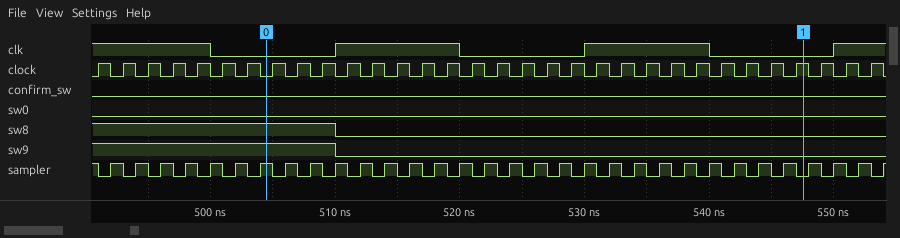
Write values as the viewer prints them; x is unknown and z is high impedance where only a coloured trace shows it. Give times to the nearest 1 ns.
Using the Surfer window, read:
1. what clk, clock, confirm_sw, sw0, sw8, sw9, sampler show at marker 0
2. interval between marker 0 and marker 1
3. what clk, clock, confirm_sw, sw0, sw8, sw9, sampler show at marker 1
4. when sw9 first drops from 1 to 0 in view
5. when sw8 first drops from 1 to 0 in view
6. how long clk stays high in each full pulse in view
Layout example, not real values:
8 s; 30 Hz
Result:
clk=0, clock=0, confirm_sw=0, sw0=0, sw8=1, sw9=1, sampler=1; 43 ns; clk=0, clock=1, confirm_sw=0, sw0=0, sw8=0, sw9=0, sampler=0; 510 ns; 510 ns; 10 ns, 10 ns
